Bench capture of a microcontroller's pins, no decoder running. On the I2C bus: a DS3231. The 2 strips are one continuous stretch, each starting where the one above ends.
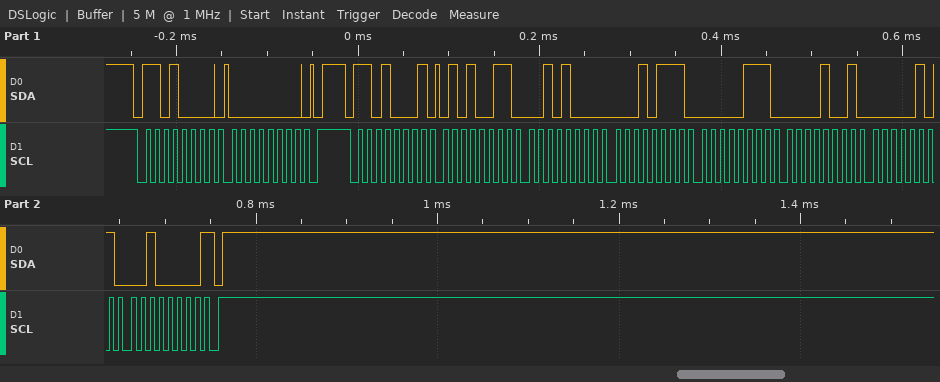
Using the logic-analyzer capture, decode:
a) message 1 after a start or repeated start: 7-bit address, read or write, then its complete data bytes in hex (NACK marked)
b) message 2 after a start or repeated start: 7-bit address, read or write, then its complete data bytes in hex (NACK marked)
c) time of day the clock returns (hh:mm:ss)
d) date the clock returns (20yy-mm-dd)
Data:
0x68 write: 00
0x68 read: 53 28 17 07 09 05 20 NACK
17:28:53
2020-05-09
